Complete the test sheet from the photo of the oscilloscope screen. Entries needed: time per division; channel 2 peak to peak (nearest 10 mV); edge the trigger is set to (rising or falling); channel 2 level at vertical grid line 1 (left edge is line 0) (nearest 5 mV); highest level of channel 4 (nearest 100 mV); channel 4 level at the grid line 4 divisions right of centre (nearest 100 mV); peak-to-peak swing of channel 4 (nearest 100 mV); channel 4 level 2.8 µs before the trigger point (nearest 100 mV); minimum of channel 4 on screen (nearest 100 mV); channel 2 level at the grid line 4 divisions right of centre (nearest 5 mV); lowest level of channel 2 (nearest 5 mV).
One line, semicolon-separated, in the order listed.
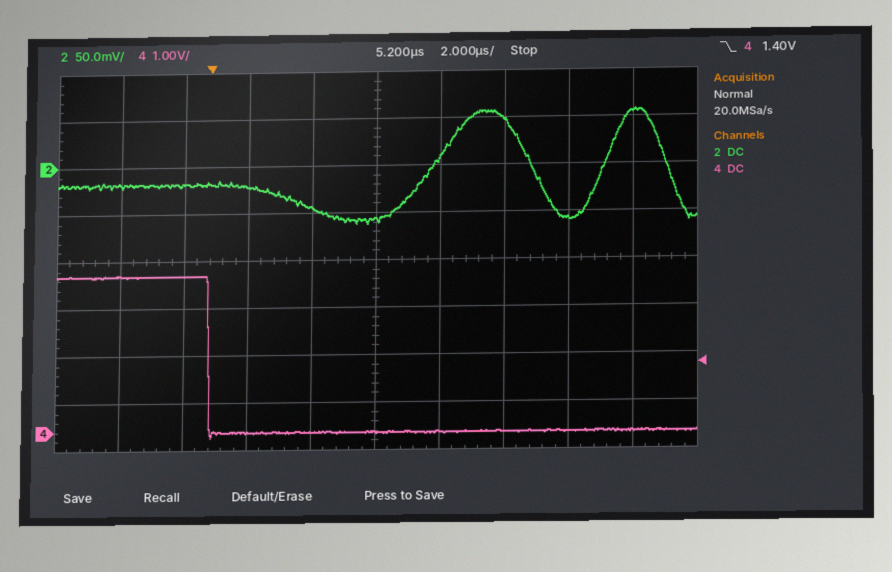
2 µs; 120 mV; falling; -20 mV; 3.3 V; 0.0 V; 3.4 V; 3.3 V; -100 mV; 55 mV; -60 mV
